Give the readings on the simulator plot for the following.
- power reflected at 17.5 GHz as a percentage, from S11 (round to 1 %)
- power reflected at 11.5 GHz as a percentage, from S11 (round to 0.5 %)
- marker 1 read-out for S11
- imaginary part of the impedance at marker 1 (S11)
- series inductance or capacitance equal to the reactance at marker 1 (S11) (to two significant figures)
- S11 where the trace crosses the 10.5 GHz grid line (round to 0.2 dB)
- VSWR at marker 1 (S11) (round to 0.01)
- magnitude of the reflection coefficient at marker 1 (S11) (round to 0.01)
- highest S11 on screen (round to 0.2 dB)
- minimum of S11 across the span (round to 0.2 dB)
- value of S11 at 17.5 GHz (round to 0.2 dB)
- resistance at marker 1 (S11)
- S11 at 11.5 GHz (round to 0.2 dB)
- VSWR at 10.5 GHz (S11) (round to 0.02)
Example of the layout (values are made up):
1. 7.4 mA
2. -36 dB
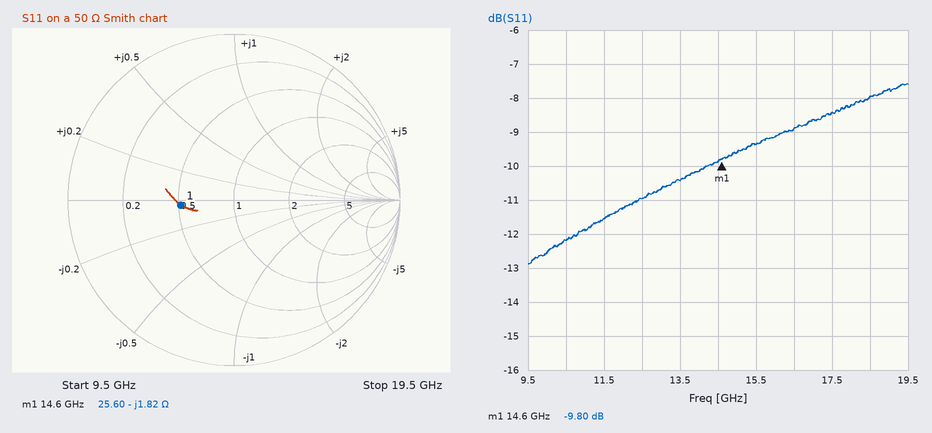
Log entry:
1. 14 %
2. 7.0 %
3. -9.80 dB
4. -1.82 Ω
5. 6.0 pF
6. -12.2 dB
7. 1.96
8. 0.32
9. -7.6 dB
10. -12.8 dB
11. -8.4 dB
12. 25.60 Ω
13. -11.6 dB
14. 1.66
